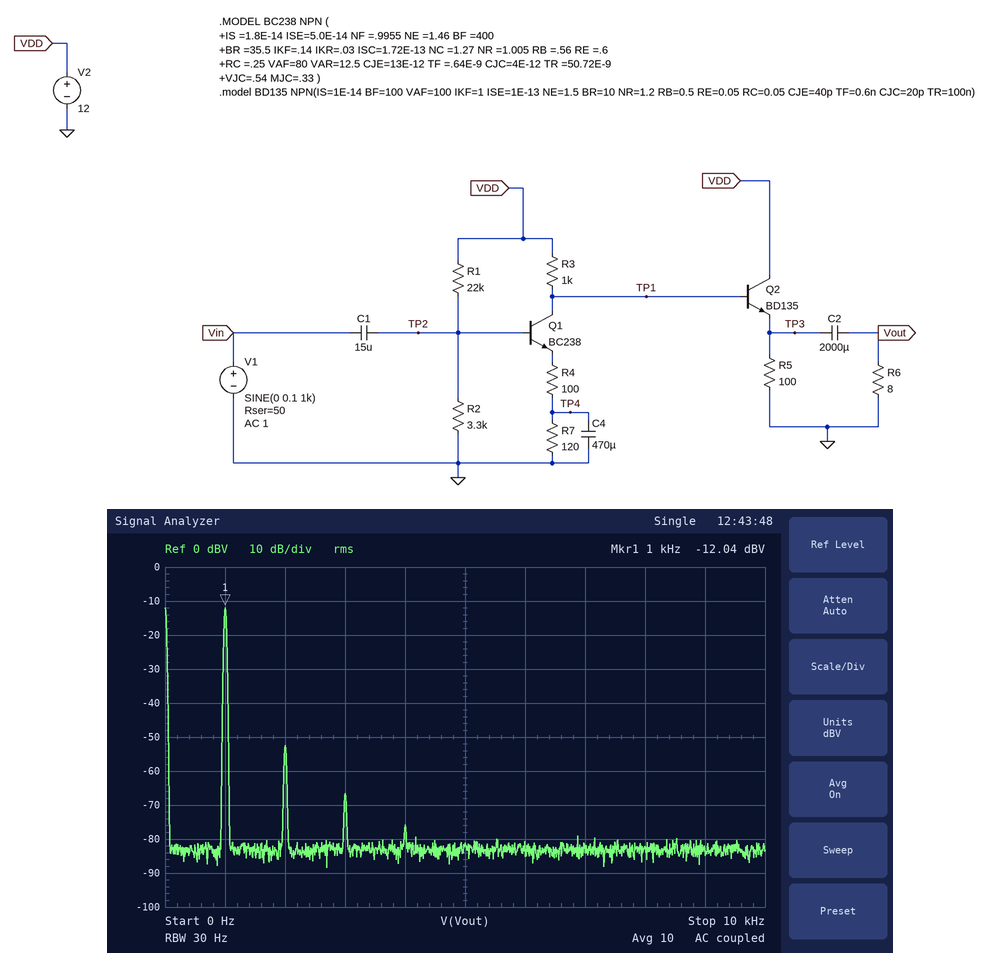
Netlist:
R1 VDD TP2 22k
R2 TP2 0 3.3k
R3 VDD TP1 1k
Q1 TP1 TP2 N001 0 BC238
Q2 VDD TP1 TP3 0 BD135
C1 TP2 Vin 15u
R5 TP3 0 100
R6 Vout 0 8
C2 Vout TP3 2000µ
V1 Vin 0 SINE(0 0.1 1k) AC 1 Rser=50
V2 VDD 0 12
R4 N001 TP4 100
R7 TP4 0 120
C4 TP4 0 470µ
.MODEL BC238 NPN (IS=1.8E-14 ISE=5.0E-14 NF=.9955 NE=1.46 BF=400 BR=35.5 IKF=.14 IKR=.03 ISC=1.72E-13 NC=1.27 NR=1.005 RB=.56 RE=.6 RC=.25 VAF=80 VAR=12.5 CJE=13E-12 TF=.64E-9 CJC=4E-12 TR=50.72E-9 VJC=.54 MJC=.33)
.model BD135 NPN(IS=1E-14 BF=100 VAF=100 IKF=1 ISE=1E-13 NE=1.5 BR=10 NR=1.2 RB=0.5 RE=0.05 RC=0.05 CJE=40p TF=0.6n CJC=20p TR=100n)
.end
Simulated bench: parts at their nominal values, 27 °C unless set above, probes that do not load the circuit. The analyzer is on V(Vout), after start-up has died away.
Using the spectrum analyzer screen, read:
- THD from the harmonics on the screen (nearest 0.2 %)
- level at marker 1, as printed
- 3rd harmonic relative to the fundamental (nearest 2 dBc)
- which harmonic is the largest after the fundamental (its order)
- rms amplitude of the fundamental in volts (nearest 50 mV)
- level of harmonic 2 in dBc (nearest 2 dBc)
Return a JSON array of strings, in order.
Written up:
["1.0 %", "-12.04 dBV", "-54 dBc", "2", "250 mV", "-40 dBc"]
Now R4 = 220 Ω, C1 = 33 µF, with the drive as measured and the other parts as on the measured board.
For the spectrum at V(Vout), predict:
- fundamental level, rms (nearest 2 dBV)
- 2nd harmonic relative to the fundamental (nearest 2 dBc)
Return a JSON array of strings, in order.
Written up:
["-18 dBV", "-44 dBc"]
